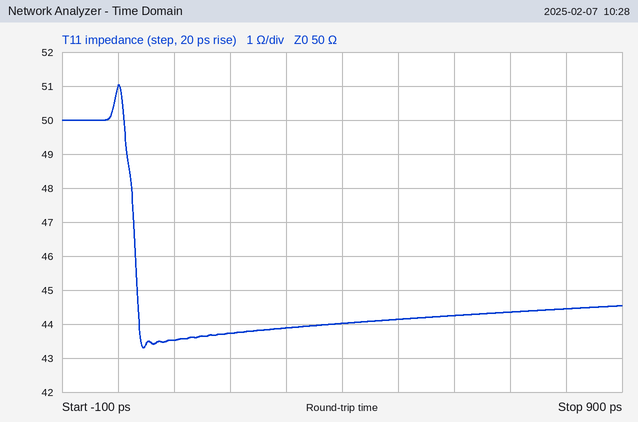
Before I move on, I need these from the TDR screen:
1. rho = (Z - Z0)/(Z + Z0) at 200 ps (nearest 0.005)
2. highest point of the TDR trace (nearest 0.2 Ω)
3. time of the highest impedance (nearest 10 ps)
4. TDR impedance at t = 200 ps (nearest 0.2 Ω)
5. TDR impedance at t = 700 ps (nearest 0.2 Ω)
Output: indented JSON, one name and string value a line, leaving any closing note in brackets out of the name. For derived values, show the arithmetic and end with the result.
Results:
{
  "rho = (Z - Z0)/(Z + Z0) at 200 ps": "(43.8 − 50)/(43.8 + 50) ≈ -0.0661, so -0.065 to the nearest 0.005",
  "highest point of the TDR trace": "51.0 Ω",
  "time of the highest impedance": "0 ps",
  "TDR impedance at t = 200 ps": "43.8 Ω",
  "TDR impedance at t = 700 ps": "44.4 Ω"
}
